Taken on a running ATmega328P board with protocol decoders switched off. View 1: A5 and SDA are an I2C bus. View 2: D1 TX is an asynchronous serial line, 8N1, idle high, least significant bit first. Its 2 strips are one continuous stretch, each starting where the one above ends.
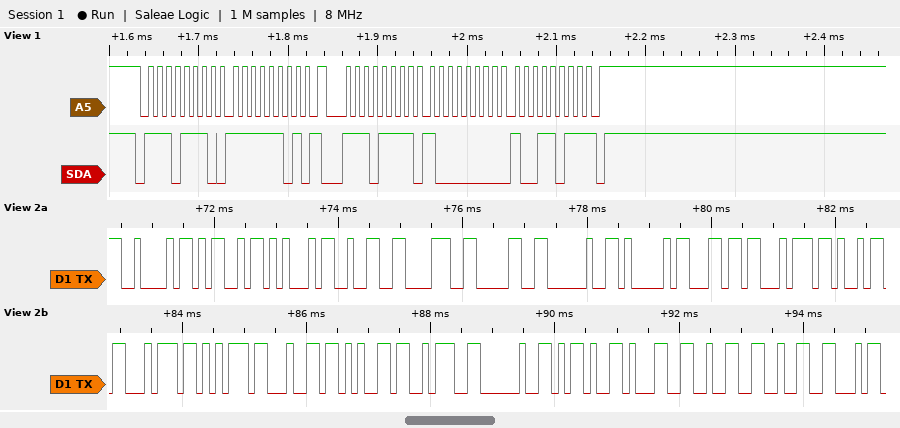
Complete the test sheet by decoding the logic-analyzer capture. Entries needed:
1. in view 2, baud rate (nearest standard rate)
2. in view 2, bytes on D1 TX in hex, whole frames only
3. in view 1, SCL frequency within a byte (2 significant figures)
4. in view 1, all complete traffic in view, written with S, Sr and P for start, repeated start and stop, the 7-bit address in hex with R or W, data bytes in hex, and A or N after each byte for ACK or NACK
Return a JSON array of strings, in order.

["9600 baud", "42 4D 45 32 38 30 20 41 6C 74 69 74 75 64 65 3A 20 2D 31 32 32", "100 kHz", "S 77W A FD A Sr 77R A 80 A 9B N P"]
